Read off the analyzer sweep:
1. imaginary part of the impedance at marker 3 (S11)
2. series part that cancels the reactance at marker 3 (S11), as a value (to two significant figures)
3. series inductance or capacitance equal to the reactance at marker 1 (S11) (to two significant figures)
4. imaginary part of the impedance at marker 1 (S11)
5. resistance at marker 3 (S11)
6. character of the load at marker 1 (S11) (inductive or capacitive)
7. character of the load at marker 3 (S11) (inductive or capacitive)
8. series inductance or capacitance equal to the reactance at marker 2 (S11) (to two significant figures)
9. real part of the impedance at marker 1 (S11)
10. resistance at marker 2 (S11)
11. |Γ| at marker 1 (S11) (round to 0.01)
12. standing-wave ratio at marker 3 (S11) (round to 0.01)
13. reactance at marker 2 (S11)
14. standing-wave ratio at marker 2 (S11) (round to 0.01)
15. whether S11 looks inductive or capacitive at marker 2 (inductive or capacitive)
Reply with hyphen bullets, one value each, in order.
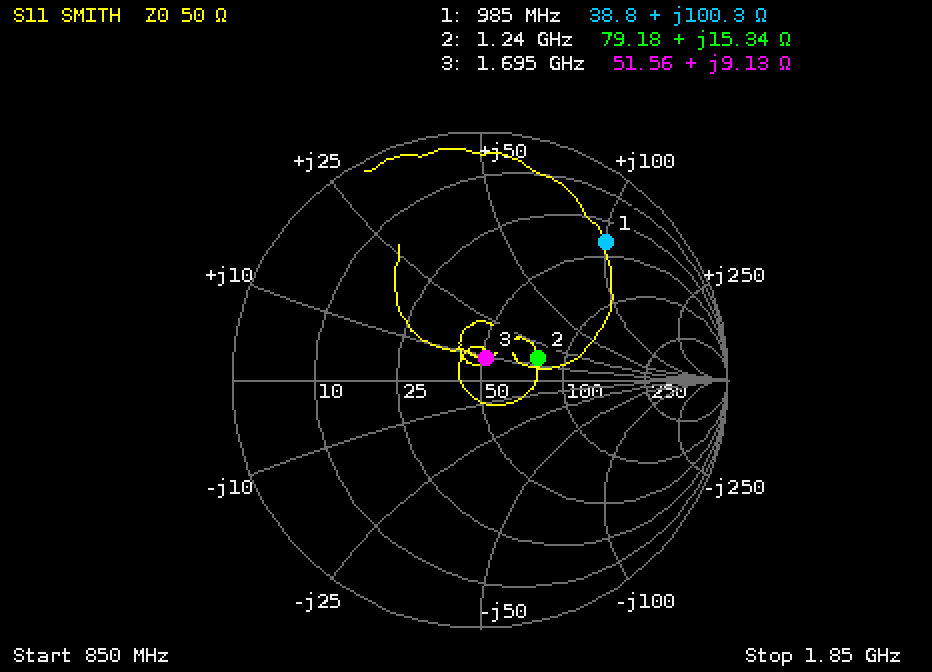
- +9.13 Ω
- 10 pF
- 16 nH
- +100.3 Ω
- 51.56 Ω
- inductive
- inductive
- 2.0 nH
- 38.8 Ω
- 79.18 Ω
- 0.75
- 1.20
- +15.34 Ω
- 1.68
- inductive
